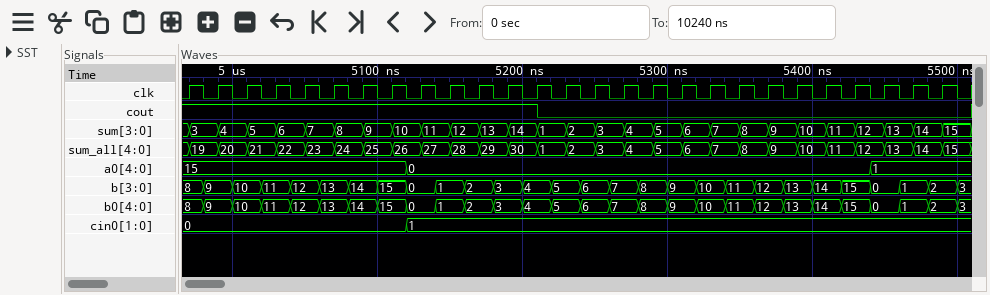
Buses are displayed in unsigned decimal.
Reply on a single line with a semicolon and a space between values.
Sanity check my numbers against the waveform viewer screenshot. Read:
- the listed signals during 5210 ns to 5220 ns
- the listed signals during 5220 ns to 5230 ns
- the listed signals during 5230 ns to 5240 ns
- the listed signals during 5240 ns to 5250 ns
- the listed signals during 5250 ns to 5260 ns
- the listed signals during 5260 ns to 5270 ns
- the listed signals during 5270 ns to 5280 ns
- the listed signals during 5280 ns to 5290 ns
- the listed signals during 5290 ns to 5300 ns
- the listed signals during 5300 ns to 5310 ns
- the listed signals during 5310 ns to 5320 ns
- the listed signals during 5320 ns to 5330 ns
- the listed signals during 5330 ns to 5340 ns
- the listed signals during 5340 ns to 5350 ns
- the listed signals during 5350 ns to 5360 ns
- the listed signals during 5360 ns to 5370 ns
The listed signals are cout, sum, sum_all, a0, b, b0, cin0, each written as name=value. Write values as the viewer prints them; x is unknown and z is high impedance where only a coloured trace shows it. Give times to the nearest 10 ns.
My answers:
cout=0, sum=1, sum_all=1, a0=0, b=4, b0=4, cin0=1; cout=0, sum=1, sum_all=1, a0=0, b=5, b0=5, cin0=1; cout=0, sum=2, sum_all=2, a0=0, b=5, b0=5, cin0=1; cout=0, sum=2, sum_all=2, a0=0, b=6, b0=6, cin0=1; cout=0, sum=3, sum_all=3, a0=0, b=6, b0=6, cin0=1; cout=0, sum=3, sum_all=3, a0=0, b=7, b0=7, cin0=1; cout=0, sum=4, sum_all=4, a0=0, b=7, b0=7, cin0=1; cout=0, sum=4, sum_all=4, a0=0, b=8, b0=8, cin0=1; cout=0, sum=5, sum_all=5, a0=0, b=8, b0=8, cin0=1; cout=0, sum=5, sum_all=5, a0=0, b=9, b0=9, cin0=1; cout=0, sum=6, sum_all=6, a0=0, b=9, b0=9, cin0=1; cout=0, sum=6, sum_all=6, a0=0, b=10, b0=10, cin0=1; cout=0, sum=7, sum_all=7, a0=0, b=10, b0=10, cin0=1; cout=0, sum=7, sum_all=7, a0=0, b=11, b0=11, cin0=1; cout=0, sum=8, sum_all=8, a0=0, b=11, b0=11, cin0=1; cout=0, sum=8, sum_all=8, a0=0, b=12, b0=12, cin0=1
